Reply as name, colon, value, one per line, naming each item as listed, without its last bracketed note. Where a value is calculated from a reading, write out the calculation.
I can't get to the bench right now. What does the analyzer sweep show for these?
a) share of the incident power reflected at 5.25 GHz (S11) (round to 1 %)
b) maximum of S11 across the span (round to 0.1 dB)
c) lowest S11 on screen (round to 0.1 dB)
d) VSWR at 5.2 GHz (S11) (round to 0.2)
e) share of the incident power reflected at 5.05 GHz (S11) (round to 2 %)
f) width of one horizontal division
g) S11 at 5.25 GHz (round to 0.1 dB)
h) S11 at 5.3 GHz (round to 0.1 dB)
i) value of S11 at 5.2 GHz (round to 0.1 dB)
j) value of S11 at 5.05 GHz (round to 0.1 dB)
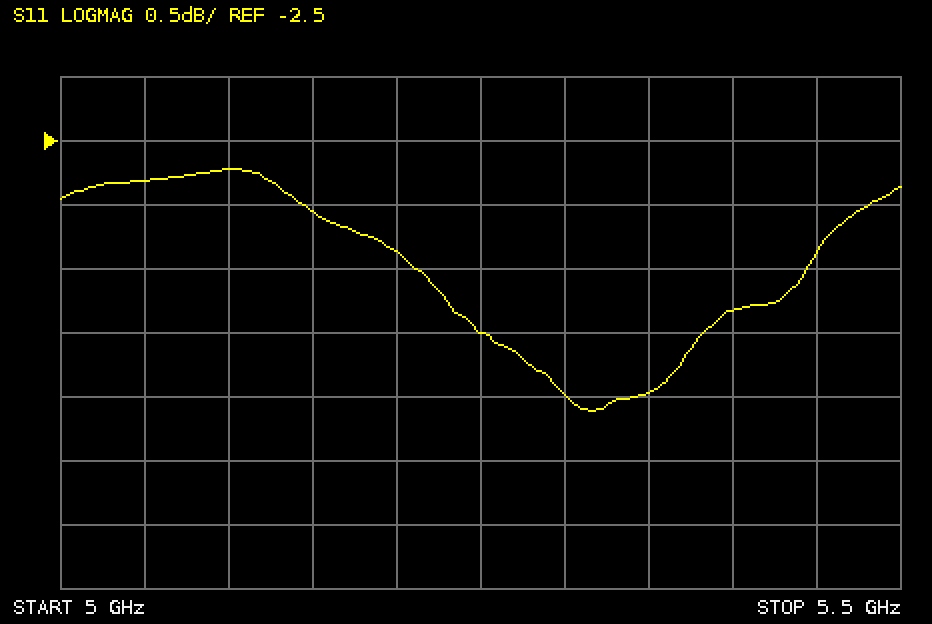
share of the incident power reflected at 5.25 GHz (S11): 10^(-4/10) ≈ 40 %
maximum of S11 across the span: -2.7 dB
lowest S11 on screen: -4.6 dB
VSWR at 5.2 GHz (S11): |Γ| = 10^(-3.4/20) = 0.6761; VSWR = (1 + 0.6761)/(1 − 0.6761) ≈ 5.2
share of the incident power reflected at 5.05 GHz (S11): 10^(-2.8/10) ≈ 52 %
width of one horizontal division: 50 MHz
S11 at 5.25 GHz: -4.0 dB
S11 at 5.3 GHz: -4.5 dB
value of S11 at 5.2 GHz: -3.4 dB
value of S11 at 5.05 GHz: -2.8 dB
